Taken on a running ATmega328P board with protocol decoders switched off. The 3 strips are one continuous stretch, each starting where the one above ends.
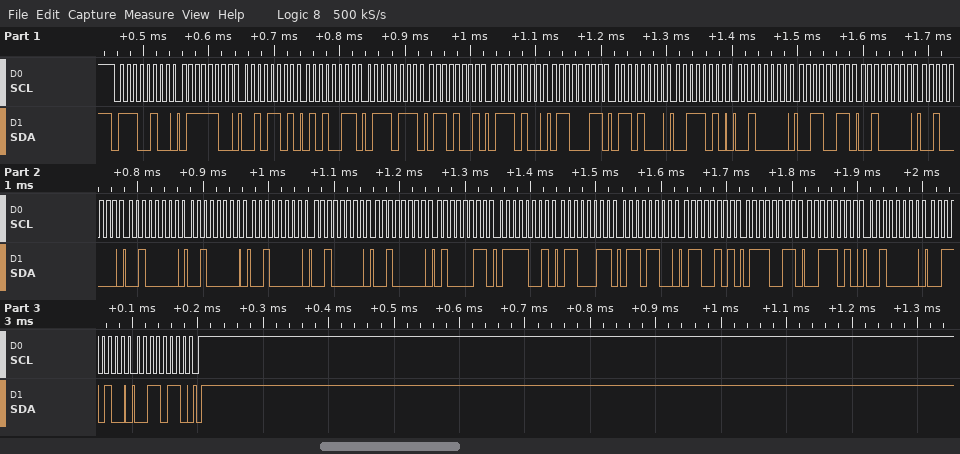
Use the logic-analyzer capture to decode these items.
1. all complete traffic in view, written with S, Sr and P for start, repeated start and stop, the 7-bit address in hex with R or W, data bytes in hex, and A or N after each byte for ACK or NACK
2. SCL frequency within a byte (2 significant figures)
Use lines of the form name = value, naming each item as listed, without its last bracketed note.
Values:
all complete traffic in view, written with S, Sr and P for start, repeated start and stop, the 7-bit address in hex with R or W, data bytes in hex, and A or N after each byte for ACK or NACK = S 72W A 7C A 2D A 53 A 77 A 69 A 74 A 63 A 68 A 3A A 20 A 33 A 20 A 20 A 20 A 20 A 20 A 20 A 20 A 43 A 79 A 63 A 6C A 65 A 73 A 3A A 20 A 34 A 36 A P
SCL frequency within a byte = 100 kHz
